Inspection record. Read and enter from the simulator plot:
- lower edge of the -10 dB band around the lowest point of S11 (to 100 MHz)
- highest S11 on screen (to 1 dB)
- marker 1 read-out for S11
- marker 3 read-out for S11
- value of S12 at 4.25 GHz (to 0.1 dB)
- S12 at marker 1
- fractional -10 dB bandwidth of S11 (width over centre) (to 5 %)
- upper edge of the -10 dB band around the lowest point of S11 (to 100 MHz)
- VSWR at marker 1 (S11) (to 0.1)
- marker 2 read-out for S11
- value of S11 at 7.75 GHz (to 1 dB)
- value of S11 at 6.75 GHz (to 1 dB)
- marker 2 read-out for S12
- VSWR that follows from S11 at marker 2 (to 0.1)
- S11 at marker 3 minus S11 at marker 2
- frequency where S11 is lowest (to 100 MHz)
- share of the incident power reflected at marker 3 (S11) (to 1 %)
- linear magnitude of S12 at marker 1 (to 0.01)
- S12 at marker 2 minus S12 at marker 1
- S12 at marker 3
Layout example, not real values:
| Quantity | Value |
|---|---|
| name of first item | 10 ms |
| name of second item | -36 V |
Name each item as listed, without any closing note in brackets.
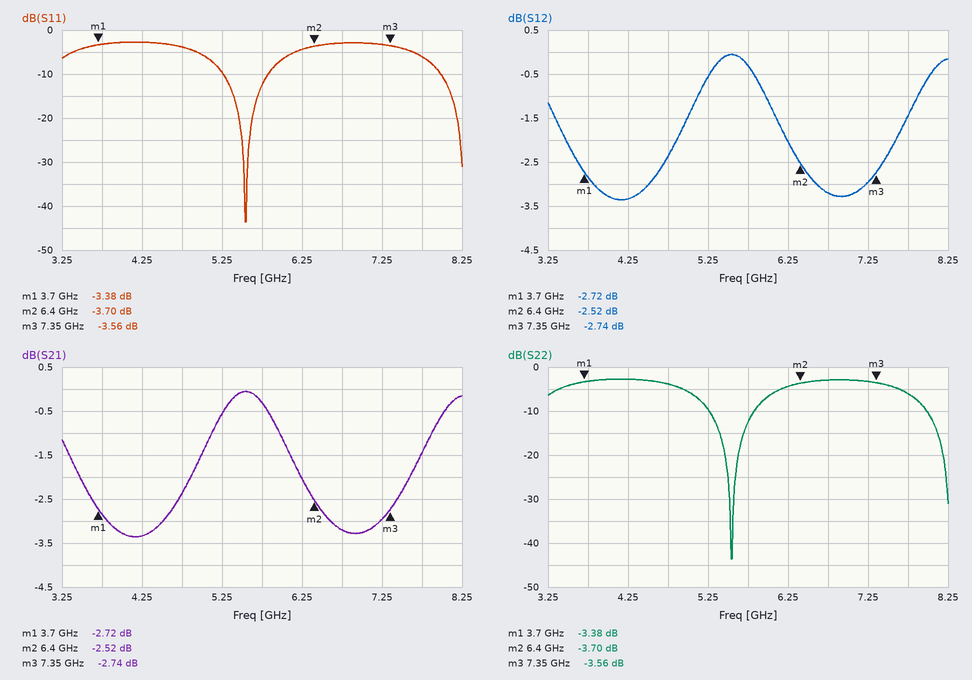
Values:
| Quantity | Value |
|---|---|
| lower edge of the -10 dB band around the lowest point of S11 | 5.3 GHz |
| highest S11 on screen | -3 dB |
| marker 1 read-out for S11 | -3.38 dB |
| marker 3 read-out for S11 | -3.56 dB |
| value of S12 at 4.25 GHz | -3.3 dB |
| S12 at marker 1 | -2.72 dB |
| fractional -10 dB bandwidth of S11 (width over centre) | 10 % |
| upper edge of the -10 dB band around the lowest point of S11 | 5.8 GHz |
| VSWR at marker 1 (S11) | 5.2 |
| marker 2 read-out for S11 | -3.70 dB |
| value of S11 at 7.75 GHz | -6 dB |
| value of S11 at 6.75 GHz | -3 dB |
| marker 2 read-out for S12 | -2.52 dB |
| VSWR that follows from S11 at marker 2 | 4.8 |
| S11 at marker 3 minus S11 at marker 2 | 0.14 dB |
| frequency where S11 is lowest | 5.5 GHz |
| share of the incident power reflected at marker 3 (S11) | 44 % |
| linear magnitude of S12 at marker 1 | 0.73 |
| S12 at marker 2 minus S12 at marker 1 | 0.20 dB |
| S12 at marker 3 | -2.74 dB |
